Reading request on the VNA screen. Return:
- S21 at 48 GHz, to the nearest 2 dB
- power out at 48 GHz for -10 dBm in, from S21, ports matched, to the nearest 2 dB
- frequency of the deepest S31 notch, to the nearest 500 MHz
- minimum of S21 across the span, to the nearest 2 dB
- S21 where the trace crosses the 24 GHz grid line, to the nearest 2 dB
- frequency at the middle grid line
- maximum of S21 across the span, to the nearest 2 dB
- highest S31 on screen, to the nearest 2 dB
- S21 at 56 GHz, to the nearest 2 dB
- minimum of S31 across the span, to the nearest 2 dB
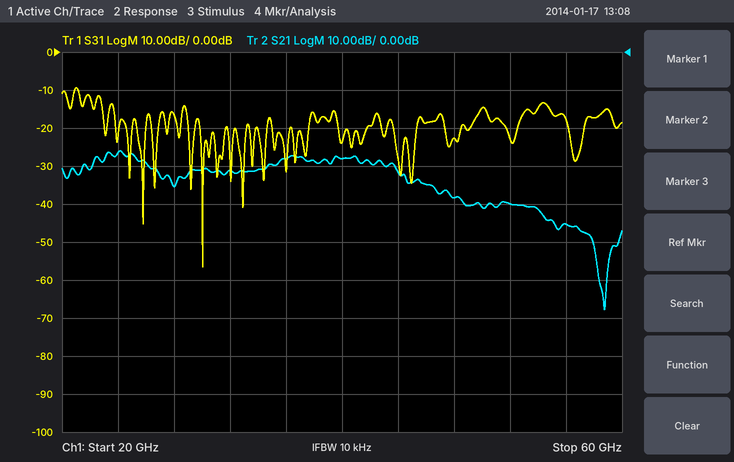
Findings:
-38 dB
-48 dBm
30.0 GHz
-68 dB
-26 dB
40 GHz
-26 dB
-10 dB
-46 dB
-56 dB
